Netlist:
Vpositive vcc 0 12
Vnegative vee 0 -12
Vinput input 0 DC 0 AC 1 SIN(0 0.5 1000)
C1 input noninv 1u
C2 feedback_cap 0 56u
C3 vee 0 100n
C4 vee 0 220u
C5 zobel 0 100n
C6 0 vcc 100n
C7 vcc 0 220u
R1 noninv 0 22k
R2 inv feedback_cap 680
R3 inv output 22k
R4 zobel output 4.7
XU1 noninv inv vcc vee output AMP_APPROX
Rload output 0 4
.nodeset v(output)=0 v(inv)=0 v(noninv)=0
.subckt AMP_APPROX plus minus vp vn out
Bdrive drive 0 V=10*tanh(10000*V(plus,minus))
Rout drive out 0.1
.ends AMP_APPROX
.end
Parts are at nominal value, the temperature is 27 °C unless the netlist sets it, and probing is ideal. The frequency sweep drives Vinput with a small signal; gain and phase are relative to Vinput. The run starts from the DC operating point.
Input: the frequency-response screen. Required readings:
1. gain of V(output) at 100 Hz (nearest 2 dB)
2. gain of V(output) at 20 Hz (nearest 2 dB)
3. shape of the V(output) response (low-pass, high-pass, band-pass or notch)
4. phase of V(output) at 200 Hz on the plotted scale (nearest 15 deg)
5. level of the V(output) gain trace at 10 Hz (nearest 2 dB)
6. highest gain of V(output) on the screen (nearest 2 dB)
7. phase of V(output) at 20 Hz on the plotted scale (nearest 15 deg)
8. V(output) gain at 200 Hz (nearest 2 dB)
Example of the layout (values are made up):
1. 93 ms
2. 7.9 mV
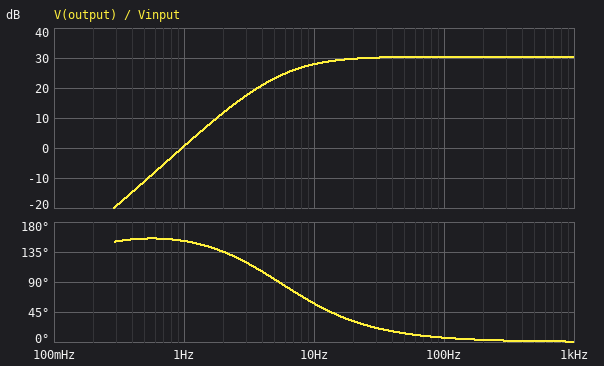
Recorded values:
1. 30 dB
2. 30 dB
3. high-pass
4. 0 deg
5. 28 dB
6. 30 dB
7. 30 deg
8. 30 dB
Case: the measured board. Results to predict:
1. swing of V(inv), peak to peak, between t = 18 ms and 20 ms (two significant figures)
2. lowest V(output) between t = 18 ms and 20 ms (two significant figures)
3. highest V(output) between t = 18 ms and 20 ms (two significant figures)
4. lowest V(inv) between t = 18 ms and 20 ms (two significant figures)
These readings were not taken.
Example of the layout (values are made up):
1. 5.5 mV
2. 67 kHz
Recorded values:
1. 590 mV
2. -9.8 V
3. 9.8 V
4. -290 mV
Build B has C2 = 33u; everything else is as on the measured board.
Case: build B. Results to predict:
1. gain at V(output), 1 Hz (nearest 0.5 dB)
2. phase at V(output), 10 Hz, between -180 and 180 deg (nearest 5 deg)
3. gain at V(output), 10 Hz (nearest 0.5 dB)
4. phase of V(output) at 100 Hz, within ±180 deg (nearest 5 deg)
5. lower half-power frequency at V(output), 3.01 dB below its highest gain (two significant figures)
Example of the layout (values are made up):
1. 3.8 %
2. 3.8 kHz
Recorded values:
1. -3.5 dB
2. 70 deg
3. 27.0 dB
4. 10 deg
5. 11 Hz
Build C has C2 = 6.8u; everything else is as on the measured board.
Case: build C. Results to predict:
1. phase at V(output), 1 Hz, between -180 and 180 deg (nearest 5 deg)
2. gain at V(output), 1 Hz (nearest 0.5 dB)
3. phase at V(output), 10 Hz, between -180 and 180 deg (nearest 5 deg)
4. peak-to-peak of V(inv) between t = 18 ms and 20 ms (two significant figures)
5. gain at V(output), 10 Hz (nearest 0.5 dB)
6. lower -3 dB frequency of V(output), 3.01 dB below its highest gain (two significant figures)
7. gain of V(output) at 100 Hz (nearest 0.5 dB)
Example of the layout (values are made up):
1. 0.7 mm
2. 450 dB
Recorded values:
1. 125 deg
2. -14.5 dB
3. 105 deg
4. 600 mV
5. 17.5 dB
6. 36 Hz
7. 30.0 dB
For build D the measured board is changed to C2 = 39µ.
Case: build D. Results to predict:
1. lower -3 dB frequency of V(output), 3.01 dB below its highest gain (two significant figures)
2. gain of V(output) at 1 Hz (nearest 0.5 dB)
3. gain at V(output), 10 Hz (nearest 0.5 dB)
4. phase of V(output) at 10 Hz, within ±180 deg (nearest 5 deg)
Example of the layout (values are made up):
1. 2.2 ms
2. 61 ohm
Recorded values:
1. 10 Hz
2. -2.5 dB
3. 27.5 dB
4. 65 deg
